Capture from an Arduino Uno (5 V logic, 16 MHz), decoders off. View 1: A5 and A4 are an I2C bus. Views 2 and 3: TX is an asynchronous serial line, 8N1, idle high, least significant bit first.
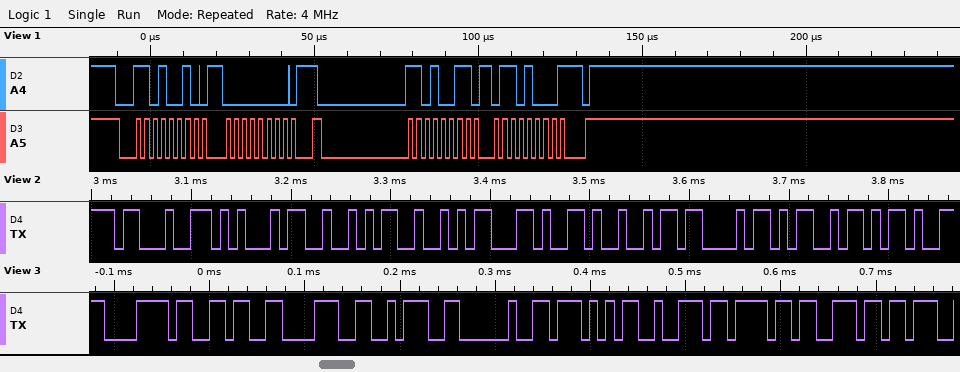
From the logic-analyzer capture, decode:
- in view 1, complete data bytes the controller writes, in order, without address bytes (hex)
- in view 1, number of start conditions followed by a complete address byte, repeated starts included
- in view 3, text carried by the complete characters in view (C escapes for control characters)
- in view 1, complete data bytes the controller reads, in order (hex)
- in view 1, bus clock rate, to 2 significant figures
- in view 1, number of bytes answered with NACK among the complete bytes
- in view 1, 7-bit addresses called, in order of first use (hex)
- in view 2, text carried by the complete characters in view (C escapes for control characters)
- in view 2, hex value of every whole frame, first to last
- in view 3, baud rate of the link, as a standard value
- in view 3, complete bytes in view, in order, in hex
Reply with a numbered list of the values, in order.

1. 00
2. 2
3. "x68: Wron"
4. 68
5. 400 kHz
6. 1
7. 0x69
8. "#ERR,ICM-"
9. 0x23 0x45 0x52 0x52 0x2C 0x49 0x43 0x4D 0x2D
10. 115200 baud
11. 0x78 0x36 0x38 0x3A 0x20 0x57 0x72 0x6F 0x6E
